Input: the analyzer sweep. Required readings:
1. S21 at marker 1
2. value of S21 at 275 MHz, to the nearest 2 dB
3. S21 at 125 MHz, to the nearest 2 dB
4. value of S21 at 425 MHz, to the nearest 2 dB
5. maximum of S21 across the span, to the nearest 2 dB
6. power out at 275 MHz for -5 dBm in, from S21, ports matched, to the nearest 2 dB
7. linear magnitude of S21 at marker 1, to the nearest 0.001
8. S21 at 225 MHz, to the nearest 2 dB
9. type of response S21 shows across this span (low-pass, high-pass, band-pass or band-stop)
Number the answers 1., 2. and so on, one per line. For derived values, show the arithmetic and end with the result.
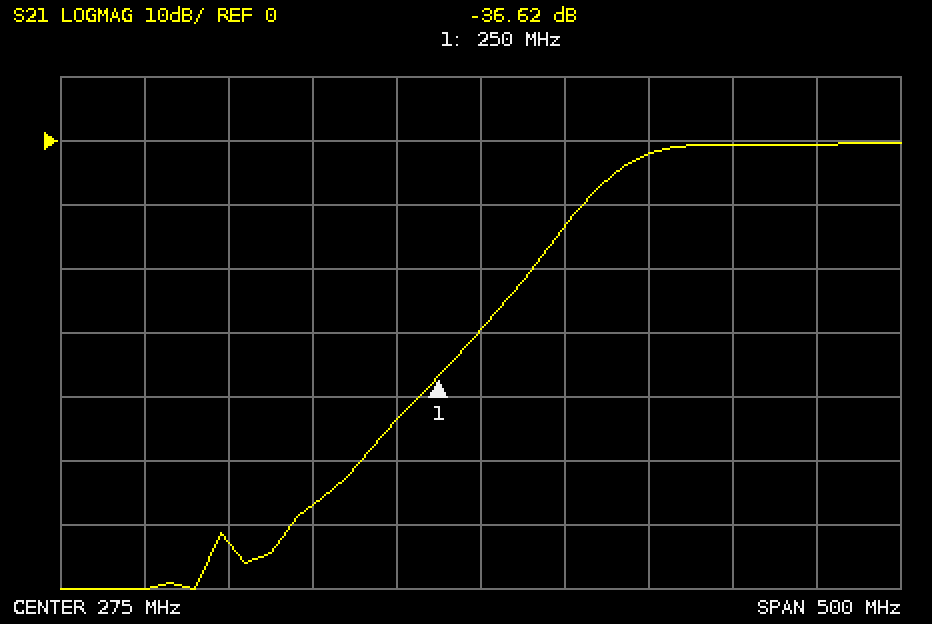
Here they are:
1. -36.62 dB
2. -30 dB
3. -62 dB
4. 0 dB
5. 0 dB
6. -5 dBm + (-30 dB) = -34 dBm
7. 10^(-36.62/20) ≈ 0.015
8. -44 dB
9. high-pass
